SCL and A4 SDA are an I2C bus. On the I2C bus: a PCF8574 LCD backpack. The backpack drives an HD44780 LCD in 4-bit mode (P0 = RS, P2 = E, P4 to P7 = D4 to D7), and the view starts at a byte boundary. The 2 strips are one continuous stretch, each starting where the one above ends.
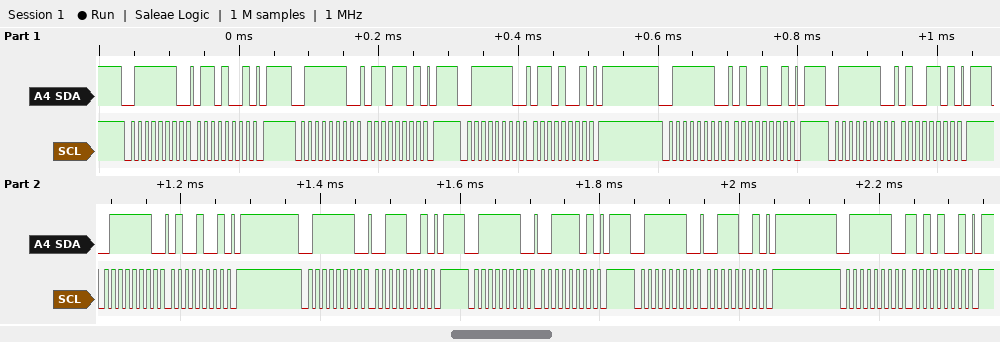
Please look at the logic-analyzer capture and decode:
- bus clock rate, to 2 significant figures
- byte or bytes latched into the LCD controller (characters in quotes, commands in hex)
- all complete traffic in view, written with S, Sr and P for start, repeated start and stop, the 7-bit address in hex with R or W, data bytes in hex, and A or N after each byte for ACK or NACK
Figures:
100 kHz
'd'
S 3FW A 69 A P S 3FW A 6D A P S 3FW A 69 A P S 3FW A 49 A P S 3FW A 4D A P S 3FW A 49 A P S 3FW A 39 A P S 3FW A 3D A P S 3FW A 39 A P S 3FW A A9 A P
